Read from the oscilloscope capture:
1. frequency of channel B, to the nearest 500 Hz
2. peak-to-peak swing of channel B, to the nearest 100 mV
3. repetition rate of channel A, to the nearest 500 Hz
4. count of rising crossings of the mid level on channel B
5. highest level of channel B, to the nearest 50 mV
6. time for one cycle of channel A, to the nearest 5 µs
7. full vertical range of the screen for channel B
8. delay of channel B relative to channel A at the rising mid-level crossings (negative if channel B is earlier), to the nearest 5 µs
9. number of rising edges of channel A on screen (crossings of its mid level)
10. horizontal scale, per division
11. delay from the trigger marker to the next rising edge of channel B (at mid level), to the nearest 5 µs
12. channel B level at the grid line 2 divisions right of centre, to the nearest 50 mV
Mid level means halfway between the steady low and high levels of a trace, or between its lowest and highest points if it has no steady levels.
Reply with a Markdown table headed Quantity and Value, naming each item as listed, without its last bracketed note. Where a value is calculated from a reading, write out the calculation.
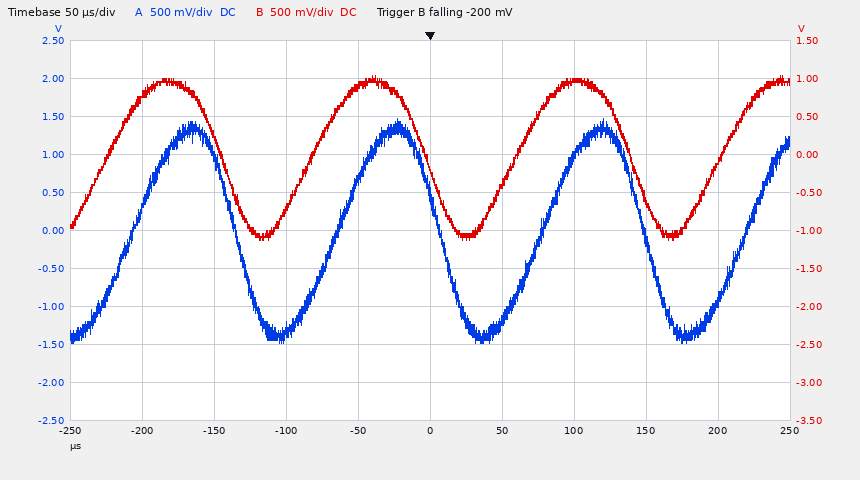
| Quantity | Value |
|---|---|
| frequency of channel B, to the nearest 500 Hz | 7.0 kHz |
| peak-to-peak swing of channel B, to the nearest 100 mV | 2.20 V |
| repetition rate of channel A, to the nearest 500 Hz | 1 / 140 µs ≈ 7.14 kHz, so 7.0 kHz to the nearest 500 Hz |
| count of rising crossings of the mid level on channel B | 4 |
| highest level of channel B, to the nearest 50 mV | 1.05 V |
| time for one cycle of channel A, to the nearest 5 µs | 140 µs |
| full vertical range of the screen for channel B | 5 V |
| delay of channel B relative to channel A at the rising mid-level crossings (negative if channel B is earlier), to the nearest 5 µs | -20 µs |
| number of rising edges of channel A on screen | 4 |
| horizontal scale, per division | 50 µs |
| delay from the trigger marker to the next rising edge of channel B (at mid level), to the nearest 5 µs | 60 µs |
| channel B level at the grid line 2 divisions right of centre, to the nearest 50 mV | 950 mV |
